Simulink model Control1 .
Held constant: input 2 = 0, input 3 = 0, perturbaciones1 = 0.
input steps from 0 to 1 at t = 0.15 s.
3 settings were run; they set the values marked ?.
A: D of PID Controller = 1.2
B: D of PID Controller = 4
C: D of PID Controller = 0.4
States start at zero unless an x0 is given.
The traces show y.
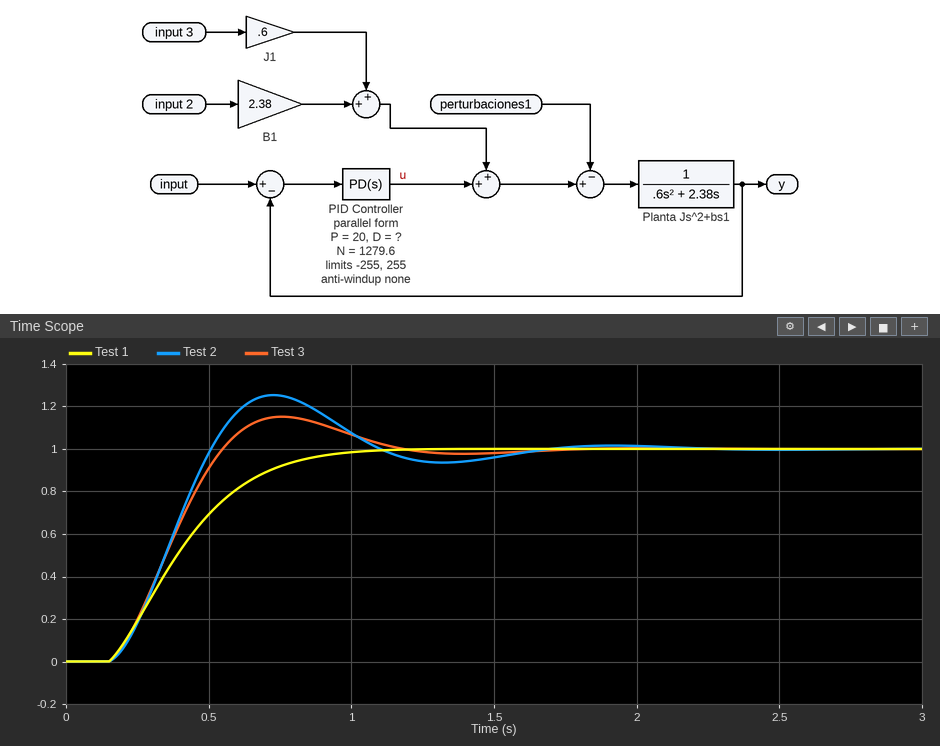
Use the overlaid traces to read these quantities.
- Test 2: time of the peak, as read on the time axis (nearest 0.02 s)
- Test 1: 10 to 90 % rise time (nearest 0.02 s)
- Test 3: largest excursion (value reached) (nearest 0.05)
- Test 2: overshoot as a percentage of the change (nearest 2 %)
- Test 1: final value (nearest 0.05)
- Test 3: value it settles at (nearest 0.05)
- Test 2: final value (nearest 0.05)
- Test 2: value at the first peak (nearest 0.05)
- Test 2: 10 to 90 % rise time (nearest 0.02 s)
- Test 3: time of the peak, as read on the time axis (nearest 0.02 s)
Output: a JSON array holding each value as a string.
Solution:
["0.72 s", "0.50 s", "1.15", "26 %", "1.00", "1.00", "1.00", "1.25", "0.26 s", "0.76 s"]
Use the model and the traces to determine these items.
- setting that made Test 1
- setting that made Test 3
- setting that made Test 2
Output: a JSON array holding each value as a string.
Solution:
["B", "A", "C"]
